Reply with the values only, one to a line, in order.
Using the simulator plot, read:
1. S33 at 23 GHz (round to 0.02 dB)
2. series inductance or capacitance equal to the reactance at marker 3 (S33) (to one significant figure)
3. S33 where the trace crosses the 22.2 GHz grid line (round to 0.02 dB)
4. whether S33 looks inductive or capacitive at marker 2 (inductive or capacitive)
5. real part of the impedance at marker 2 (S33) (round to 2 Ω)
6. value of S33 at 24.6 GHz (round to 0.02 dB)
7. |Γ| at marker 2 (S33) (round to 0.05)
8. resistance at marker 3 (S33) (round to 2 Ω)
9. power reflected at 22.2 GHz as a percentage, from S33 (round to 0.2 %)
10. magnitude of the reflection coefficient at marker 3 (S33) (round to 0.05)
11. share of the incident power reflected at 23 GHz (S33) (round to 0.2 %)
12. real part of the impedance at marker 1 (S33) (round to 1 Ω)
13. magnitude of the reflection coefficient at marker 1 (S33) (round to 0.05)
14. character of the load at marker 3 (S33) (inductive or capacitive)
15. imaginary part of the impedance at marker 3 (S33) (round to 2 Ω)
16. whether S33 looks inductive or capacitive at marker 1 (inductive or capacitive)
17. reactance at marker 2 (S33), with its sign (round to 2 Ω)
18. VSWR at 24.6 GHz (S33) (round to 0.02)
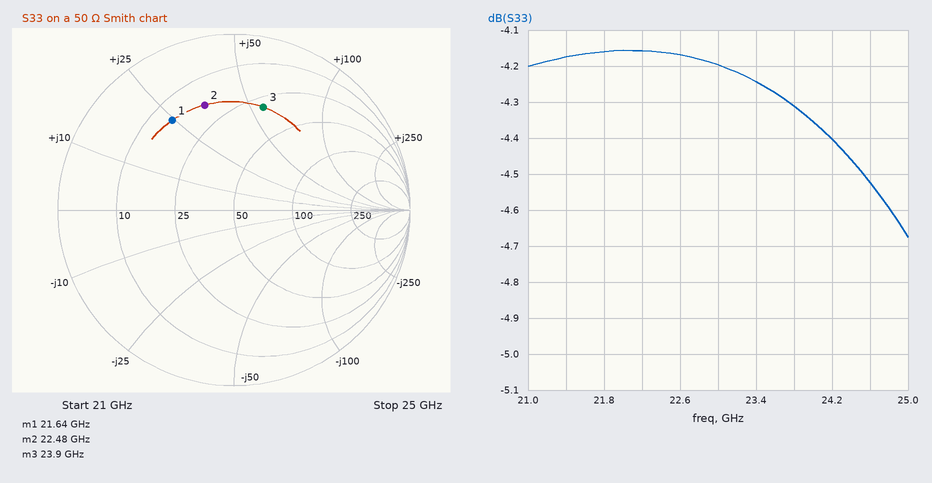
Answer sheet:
-4.20 dB
400 pH
-4.16 dB
inductive
18 Ω
-4.52 dB
0.60
30 Ω
38.4 %
0.60
38.0 %
15 Ω
0.60
inductive
+56 Ω
inductive
+34 Ω
3.92
